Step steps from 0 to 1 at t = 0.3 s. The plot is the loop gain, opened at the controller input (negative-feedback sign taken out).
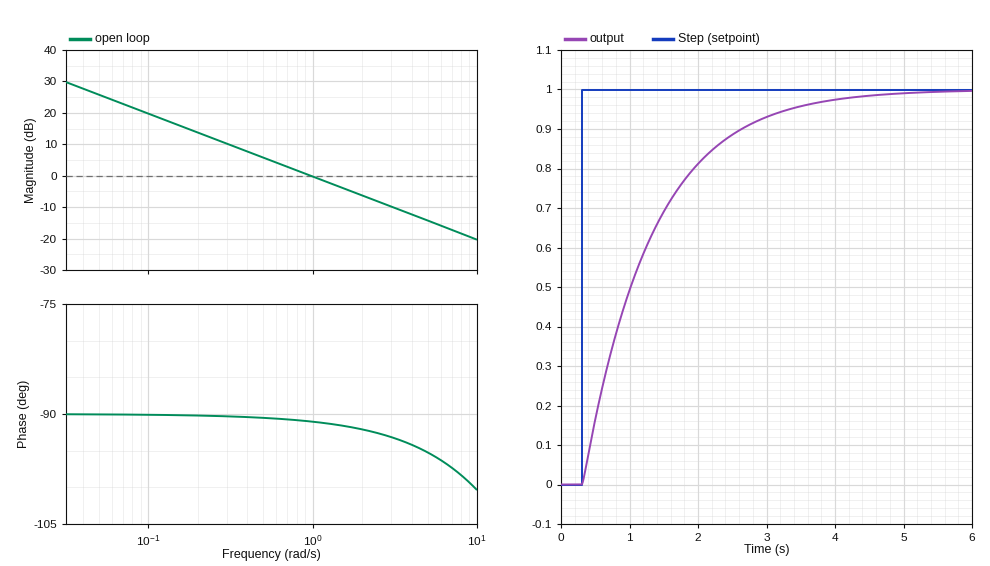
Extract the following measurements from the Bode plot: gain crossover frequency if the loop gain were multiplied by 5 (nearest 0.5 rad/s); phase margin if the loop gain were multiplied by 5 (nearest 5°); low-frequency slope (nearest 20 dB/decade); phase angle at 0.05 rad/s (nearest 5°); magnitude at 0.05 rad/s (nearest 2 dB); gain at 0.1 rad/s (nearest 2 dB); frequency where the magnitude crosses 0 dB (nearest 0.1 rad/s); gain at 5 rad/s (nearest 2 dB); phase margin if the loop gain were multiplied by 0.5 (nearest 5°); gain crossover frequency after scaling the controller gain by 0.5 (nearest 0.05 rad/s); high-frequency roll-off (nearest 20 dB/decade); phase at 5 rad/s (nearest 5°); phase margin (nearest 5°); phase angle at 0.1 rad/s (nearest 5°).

5.0 rad/s
85°
-20 dB/decade
-90°
26 dB
20 dB
1.0 rad/s
-14 dB
90°
0.50 rad/s
-20 dB/decade
-95°
90°
-90°
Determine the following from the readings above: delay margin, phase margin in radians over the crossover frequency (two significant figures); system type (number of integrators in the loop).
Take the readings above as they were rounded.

1.6 s
1
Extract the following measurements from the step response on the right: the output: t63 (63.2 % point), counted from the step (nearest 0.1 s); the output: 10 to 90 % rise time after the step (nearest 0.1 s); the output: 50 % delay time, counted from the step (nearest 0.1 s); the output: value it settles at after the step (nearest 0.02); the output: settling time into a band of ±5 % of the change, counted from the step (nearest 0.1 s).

1.0 s
2.2 s
0.7 s
1.00
3.0 s
